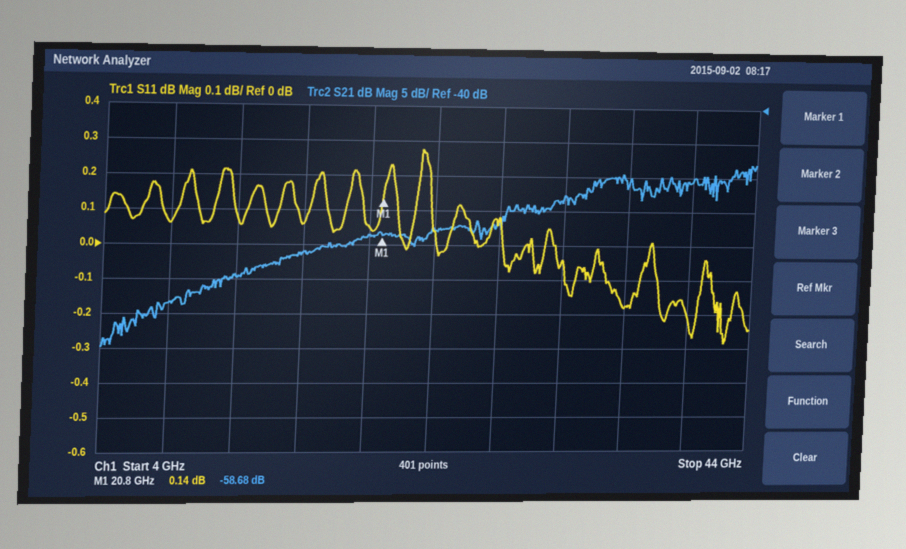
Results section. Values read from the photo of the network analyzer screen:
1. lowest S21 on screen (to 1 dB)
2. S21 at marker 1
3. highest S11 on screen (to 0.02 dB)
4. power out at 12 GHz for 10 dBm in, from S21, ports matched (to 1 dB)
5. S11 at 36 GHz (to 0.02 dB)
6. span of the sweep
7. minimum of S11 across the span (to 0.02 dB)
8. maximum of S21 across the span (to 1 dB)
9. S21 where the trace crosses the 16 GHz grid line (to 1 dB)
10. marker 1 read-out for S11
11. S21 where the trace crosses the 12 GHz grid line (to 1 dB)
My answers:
-75 dB
-58.68 dB
0.28 dB
-55 dBm
-0.18 dB
40 GHz
-0.28 dB
-48 dB
-61 dB
0.14 dB
-65 dB
